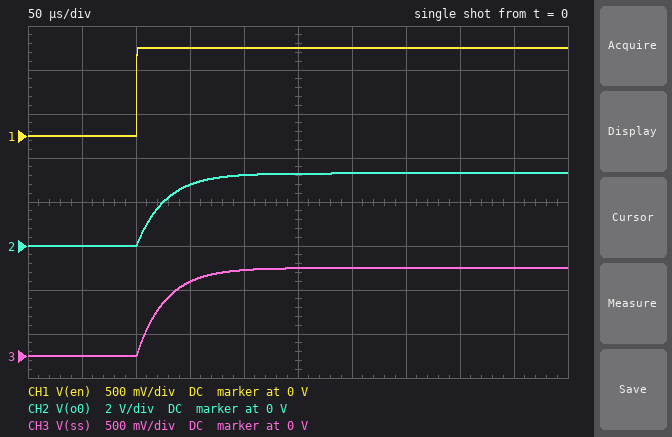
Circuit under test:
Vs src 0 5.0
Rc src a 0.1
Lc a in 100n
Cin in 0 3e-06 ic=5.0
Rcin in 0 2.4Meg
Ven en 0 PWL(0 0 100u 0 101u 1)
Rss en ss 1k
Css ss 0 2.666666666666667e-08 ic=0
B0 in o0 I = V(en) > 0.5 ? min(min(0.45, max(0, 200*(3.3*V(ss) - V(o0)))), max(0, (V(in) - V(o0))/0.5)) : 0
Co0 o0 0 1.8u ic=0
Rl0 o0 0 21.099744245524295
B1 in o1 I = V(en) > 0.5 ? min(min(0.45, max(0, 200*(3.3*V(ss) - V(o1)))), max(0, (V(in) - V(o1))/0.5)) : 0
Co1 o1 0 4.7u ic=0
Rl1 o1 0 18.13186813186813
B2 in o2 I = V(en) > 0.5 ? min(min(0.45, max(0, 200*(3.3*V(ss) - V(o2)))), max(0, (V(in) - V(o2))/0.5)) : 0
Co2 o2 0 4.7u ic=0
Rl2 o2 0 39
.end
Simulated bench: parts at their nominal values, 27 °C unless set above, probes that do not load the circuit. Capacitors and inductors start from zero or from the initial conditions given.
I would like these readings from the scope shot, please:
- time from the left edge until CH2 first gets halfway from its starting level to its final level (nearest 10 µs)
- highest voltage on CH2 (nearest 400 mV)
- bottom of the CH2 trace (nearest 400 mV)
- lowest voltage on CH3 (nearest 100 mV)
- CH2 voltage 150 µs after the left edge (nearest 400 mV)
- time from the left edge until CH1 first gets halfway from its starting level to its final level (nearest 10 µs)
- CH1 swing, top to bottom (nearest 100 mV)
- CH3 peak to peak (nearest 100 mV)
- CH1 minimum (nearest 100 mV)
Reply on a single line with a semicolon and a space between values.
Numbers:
120 µs; 3.2 V; 0 V; 0 V; 2.8 V; 100 µs; 1.0 V; 1.0 V; 0 V
